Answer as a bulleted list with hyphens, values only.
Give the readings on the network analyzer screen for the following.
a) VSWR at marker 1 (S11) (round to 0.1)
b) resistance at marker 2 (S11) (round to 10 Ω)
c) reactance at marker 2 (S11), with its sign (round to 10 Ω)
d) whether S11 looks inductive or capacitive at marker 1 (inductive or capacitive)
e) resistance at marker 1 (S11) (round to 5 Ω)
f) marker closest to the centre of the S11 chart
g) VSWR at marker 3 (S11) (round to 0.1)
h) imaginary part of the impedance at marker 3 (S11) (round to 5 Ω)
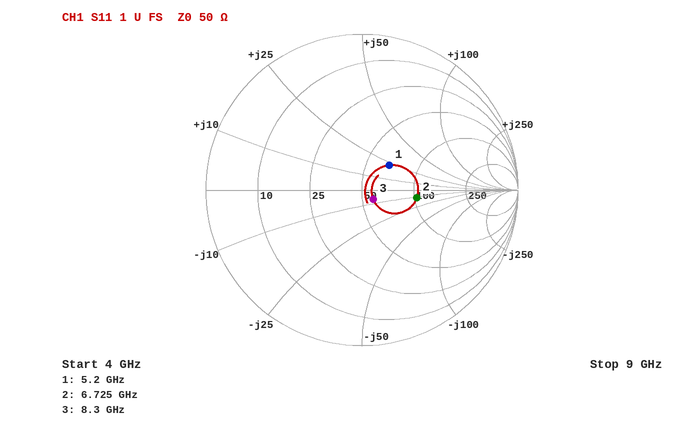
- 1.6
- 100 Ω
- -10 Ω
- inductive
- 65 Ω
- marker 3
- 1.2
- -5 Ω
